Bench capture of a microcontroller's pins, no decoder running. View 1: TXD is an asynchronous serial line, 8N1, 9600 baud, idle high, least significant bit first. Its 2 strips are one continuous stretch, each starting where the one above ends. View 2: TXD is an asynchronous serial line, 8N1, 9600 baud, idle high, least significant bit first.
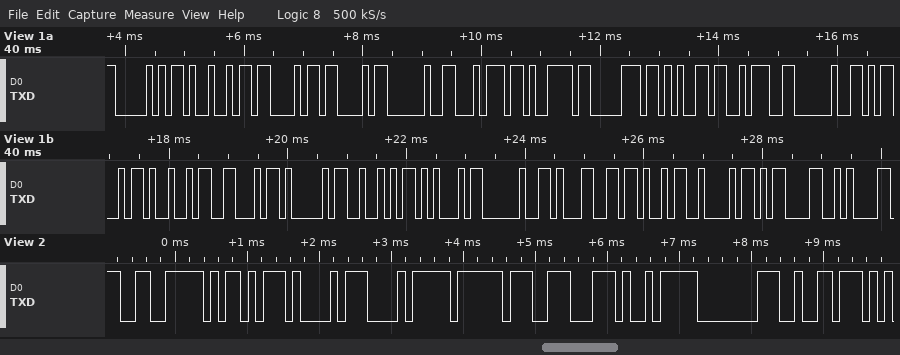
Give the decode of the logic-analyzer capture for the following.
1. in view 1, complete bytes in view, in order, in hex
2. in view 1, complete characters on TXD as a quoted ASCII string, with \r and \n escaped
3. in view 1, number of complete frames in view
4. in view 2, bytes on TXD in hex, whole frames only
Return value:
0x50 0x49 0x43 0x43 0x20 0x74 0x79 0x70 0x65 0x3A 0x20 0x4D 0x49 0x46 0x41 0x52 0x45 0x20 0x31 0x4B 0x42 0x0D 0x0A
"PICC type: MIFARE 1KB\r\n"
23
E6 AD A1 E8 BF 8E E9 80 B2
